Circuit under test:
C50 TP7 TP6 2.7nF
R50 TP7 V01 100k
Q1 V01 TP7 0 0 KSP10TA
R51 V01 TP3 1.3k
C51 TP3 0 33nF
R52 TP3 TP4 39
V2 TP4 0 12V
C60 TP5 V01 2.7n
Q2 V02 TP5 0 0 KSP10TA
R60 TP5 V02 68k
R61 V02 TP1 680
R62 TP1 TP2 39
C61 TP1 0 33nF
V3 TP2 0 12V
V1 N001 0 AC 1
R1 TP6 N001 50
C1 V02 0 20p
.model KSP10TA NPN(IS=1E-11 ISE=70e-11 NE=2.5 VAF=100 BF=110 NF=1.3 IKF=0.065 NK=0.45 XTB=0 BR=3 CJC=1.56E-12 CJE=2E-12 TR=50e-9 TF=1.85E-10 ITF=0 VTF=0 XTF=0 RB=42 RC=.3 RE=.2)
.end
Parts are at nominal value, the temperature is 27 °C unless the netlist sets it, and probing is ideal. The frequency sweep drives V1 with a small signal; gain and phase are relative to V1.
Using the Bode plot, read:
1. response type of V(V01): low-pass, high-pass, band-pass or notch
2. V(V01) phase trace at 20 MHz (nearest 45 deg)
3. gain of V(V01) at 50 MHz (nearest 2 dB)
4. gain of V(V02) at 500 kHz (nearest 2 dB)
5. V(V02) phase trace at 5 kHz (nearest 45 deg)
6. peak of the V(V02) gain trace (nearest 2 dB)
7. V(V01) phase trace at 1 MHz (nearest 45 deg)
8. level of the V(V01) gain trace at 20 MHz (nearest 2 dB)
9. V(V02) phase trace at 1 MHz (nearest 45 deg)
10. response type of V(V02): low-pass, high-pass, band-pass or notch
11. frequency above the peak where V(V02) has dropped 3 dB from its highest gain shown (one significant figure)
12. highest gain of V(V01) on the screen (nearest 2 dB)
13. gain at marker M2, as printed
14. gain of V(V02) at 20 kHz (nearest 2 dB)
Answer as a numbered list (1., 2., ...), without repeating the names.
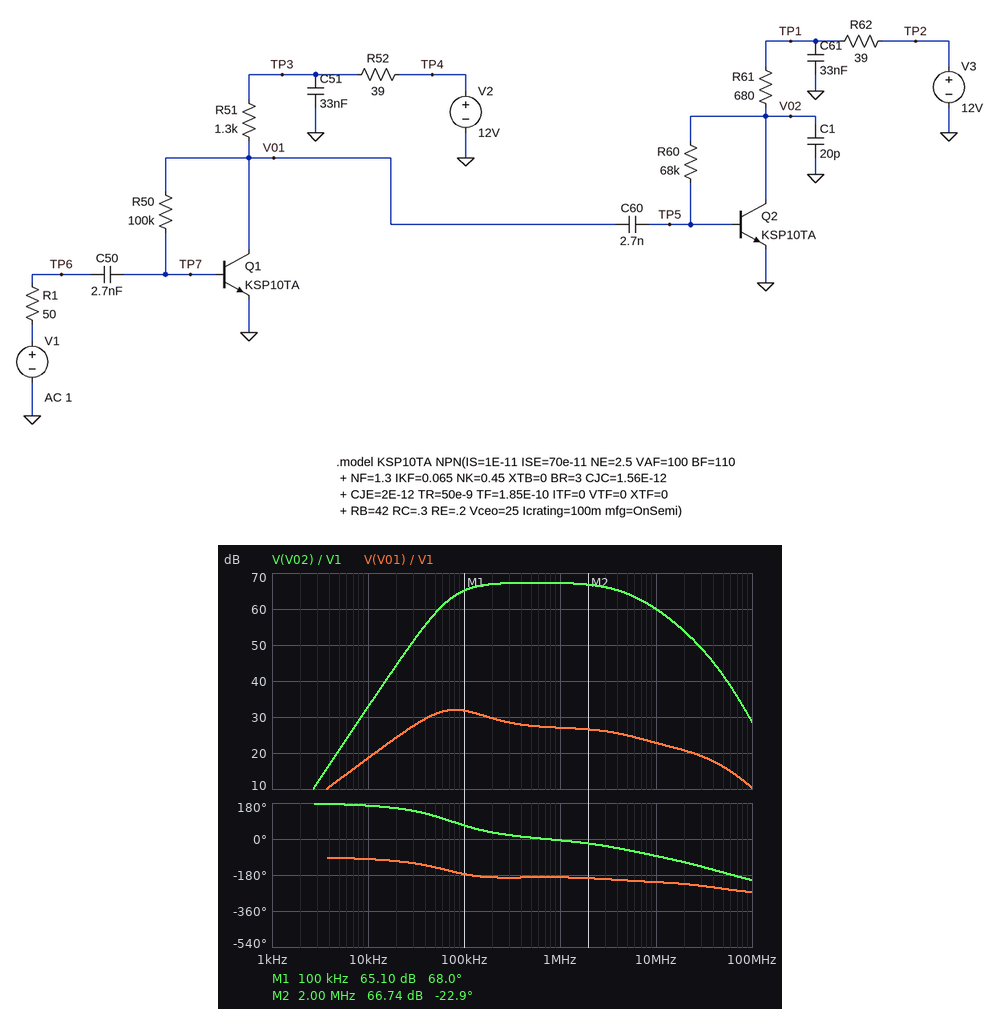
1. band-pass
2. -225 deg
3. 16 dB
4. 68 dB
5. 180 deg
6. 68 dB
7. -180 deg
8. 20 dB
9. 0 deg
10. band-pass
11. 5 MHz
12. 32 dB
13. 66.74 dB
14. 44 dB
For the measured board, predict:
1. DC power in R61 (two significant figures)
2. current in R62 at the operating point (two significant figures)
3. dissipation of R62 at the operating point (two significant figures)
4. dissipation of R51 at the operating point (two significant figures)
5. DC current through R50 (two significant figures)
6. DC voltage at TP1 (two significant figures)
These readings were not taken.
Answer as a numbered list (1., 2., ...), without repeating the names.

1. 33 mW
2. 7.0 mA
3. 1.9 mW
4. 22 mW
5. 58 µA
6. 12 V
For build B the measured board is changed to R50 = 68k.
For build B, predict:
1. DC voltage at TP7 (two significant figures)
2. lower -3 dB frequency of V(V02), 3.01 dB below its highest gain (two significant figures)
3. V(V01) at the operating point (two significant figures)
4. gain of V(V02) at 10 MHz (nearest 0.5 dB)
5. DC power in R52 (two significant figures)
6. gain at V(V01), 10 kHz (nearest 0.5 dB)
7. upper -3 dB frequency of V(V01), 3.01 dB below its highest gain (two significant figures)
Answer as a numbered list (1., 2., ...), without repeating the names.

1. 680 mV
2. 100 kHz
3. 5.3 V
4. 61.0 dB
5. 960 µW
6. 16.5 dB
7. 410 kHz
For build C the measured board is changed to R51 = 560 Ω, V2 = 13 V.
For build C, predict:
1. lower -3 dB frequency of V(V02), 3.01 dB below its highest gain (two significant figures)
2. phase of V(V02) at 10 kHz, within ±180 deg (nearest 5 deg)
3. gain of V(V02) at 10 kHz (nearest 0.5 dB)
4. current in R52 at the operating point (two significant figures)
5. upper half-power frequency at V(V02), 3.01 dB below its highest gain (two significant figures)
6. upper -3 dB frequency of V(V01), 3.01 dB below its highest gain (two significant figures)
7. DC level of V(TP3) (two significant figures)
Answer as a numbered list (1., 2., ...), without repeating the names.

1. 130 kHz
2. 170 deg
3. 29.0 dB
4. 6.5 mA
5. 5.5 MHz
6. 3.4 MHz
7. 13 V
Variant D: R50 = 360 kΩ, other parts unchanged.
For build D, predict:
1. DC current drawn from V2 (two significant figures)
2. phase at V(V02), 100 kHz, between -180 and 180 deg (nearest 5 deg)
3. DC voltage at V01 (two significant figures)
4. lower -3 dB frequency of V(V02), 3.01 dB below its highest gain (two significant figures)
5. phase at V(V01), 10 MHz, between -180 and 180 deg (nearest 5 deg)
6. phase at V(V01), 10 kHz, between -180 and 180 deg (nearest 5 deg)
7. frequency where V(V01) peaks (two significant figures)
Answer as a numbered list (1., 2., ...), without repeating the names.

1. 1.6 mA
2. 40 deg
3. 9.9 V
4. 51 kHz
5. 150 deg
6. -115 deg
7. 40 kHz
